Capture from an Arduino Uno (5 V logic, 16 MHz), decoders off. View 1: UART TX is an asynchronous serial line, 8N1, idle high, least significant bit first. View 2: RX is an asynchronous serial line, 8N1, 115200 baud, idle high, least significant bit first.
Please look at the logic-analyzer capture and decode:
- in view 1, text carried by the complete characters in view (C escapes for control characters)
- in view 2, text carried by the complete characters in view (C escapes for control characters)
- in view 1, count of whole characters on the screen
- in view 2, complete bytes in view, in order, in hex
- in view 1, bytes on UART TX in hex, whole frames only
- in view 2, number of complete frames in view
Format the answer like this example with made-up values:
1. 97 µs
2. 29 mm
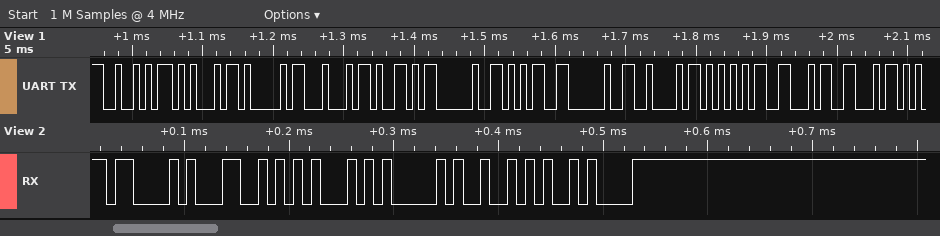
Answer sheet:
1. "READY 5 BUFF"
2. "CLEAR\n"
3. 12
4. 43 4C 45 41 52 0A
5. 0x52 0x45 0x41 0x44 0x59 0x20 0x35 0x20 0x42 0x55 0x46 0x46
6. 6
